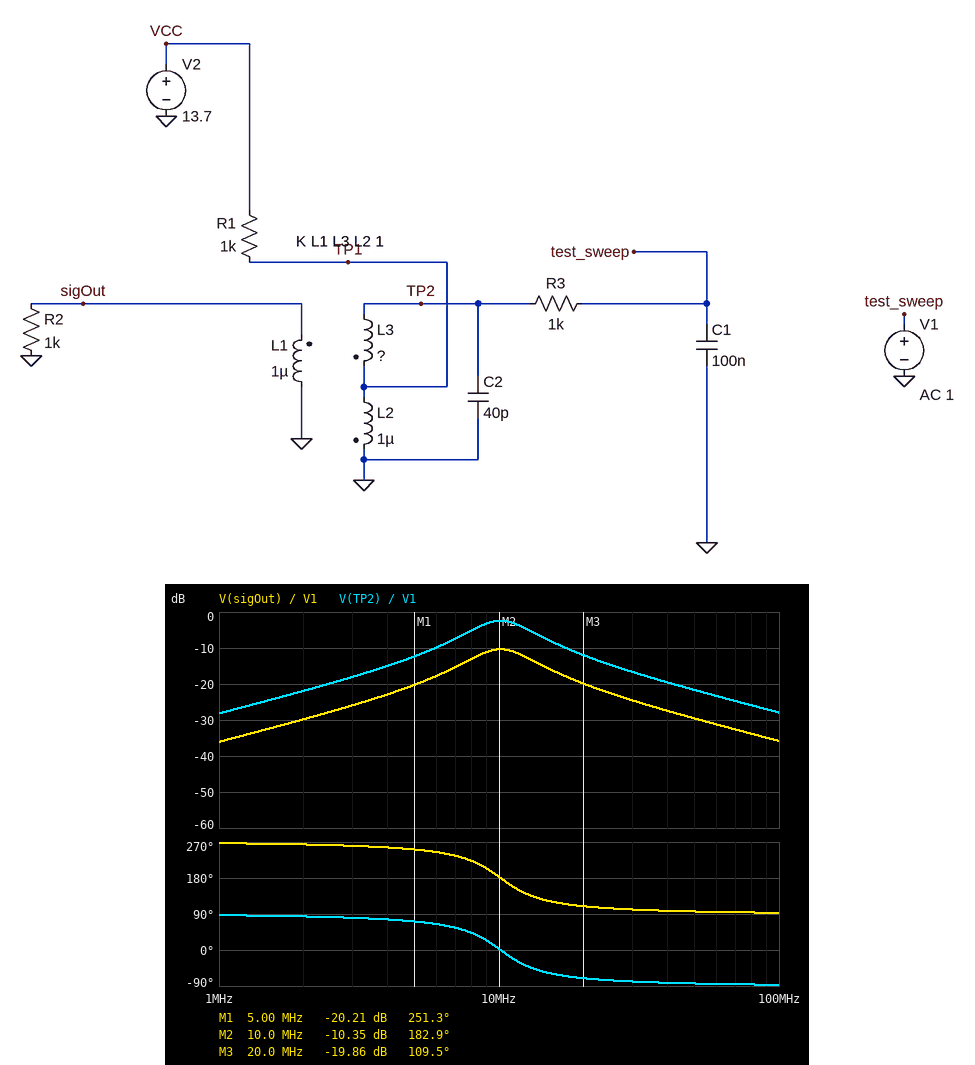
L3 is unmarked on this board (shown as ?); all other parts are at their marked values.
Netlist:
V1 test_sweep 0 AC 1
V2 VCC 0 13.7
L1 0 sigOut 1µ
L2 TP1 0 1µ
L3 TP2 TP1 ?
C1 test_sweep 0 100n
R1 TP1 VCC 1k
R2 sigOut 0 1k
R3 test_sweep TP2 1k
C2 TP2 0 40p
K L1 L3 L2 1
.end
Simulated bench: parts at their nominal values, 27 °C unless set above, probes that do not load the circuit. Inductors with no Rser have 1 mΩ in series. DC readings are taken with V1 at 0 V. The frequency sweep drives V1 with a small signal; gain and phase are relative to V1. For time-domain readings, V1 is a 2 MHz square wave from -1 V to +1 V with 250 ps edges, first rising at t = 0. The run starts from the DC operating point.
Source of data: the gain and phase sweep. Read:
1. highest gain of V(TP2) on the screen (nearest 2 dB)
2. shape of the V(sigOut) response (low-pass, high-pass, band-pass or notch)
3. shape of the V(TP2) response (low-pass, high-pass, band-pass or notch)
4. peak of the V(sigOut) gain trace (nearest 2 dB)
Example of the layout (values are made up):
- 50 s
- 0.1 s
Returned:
- -2 dB
- band-pass
- band-pass
- -10 dB
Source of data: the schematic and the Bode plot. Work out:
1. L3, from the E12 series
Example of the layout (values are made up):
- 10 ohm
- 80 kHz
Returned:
- 2.2 µH
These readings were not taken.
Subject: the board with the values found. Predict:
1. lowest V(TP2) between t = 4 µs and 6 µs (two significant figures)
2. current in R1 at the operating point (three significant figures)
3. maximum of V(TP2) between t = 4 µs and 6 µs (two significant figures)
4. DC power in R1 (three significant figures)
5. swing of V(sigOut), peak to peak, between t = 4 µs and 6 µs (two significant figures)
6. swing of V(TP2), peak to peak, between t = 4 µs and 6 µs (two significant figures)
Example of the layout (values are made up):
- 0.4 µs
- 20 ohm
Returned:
- -560 mV
- 13.7 mA
- 560 mV
- 188 mW
- 450 mV
- 1.1 V
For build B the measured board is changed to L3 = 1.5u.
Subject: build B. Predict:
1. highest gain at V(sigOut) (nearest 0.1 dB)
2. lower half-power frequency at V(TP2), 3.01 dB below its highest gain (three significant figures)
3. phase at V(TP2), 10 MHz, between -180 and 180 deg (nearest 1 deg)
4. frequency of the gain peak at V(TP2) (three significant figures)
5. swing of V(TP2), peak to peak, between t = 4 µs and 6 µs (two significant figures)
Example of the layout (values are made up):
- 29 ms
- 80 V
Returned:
- -9.9 dB
- 8.86 MHz
- 27 deg
- 11.3 MHz
- 1.0 V
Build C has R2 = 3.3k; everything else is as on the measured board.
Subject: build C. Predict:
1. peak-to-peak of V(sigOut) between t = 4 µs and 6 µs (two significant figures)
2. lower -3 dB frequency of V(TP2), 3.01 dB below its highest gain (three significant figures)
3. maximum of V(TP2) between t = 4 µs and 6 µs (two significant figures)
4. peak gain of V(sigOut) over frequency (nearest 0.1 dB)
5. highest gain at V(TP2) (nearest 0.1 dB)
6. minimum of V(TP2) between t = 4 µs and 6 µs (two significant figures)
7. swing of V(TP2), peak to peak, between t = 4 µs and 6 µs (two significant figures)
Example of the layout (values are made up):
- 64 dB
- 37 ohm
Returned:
- 470 mV
- 8.01 MHz
- 580 mV
- -9.6 dB
- -1.7 dB
- -580 mV
- 1.2 V
